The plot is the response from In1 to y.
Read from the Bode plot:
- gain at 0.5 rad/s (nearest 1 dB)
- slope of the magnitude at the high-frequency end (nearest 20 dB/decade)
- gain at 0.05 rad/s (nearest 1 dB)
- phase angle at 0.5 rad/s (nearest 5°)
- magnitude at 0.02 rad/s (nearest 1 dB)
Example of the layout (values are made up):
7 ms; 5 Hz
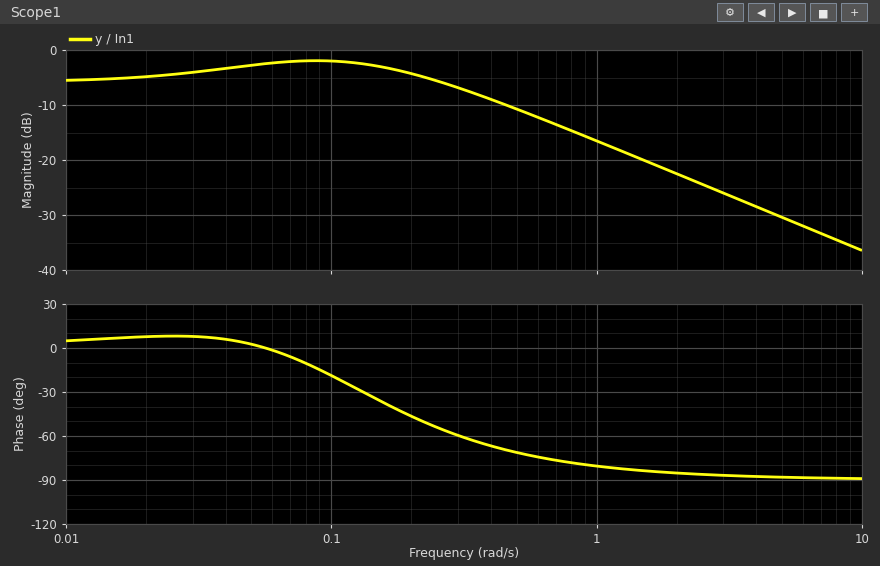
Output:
-11 dB; -20 dB/decade; -3 dB; -70°; -5 dB
